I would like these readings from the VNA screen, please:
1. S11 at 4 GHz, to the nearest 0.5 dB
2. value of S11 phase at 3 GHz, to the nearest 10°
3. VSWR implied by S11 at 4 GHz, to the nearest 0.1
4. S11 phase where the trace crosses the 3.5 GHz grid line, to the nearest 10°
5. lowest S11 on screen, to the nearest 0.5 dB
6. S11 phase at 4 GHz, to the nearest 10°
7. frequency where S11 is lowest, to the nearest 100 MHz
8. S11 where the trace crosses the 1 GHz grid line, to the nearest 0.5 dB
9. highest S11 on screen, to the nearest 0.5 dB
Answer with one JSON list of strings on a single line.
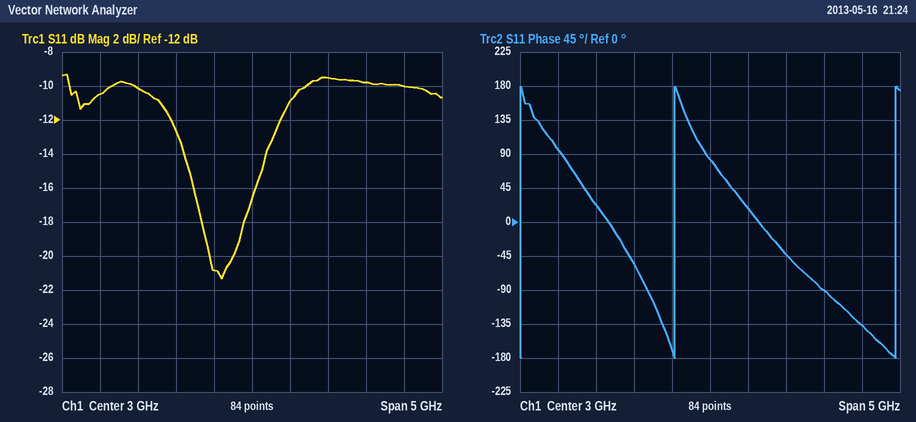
["-9.5 dB", "80°", "2.0", "20°", "-21.5 dB", "-40°", "2.6 GHz", "-10.5 dB", "-9.5 dB"]
